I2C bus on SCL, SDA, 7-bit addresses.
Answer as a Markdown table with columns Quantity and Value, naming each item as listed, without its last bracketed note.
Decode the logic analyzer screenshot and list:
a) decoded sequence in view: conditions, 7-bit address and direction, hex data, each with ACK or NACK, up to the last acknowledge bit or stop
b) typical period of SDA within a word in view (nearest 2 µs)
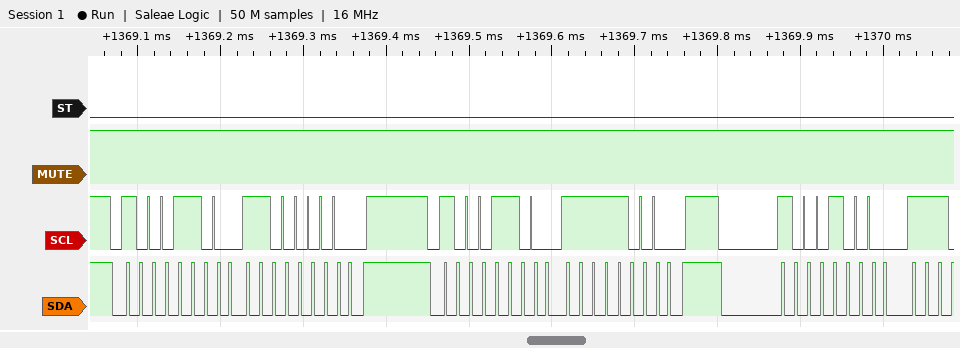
| Quantity | Value |
|---|---|
| decoded sequence in view: conditions, 7-bit address and direction, hex data, each with ACK or NACK, up to the last acknowledge bit or stop | start, address 46 write ACK, C0 ACK, stop, start, address 46 write ACK, F8 ACK, stop, start, address 44 write ACK |
| typical period of SDA within a word in view | 16 µs |
